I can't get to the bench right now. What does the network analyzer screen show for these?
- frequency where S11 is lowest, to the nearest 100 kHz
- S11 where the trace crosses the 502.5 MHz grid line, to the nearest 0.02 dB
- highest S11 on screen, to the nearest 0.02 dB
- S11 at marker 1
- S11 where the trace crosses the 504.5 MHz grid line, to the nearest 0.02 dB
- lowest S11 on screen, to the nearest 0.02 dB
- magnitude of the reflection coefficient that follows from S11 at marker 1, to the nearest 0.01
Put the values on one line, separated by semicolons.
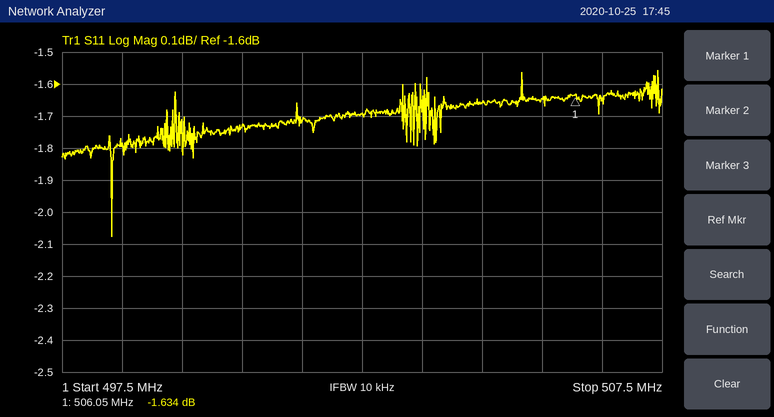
498.3 MHz; -1.70 dB; -1.56 dB; -1.634 dB; -1.66 dB; -2.08 dB; 0.83
